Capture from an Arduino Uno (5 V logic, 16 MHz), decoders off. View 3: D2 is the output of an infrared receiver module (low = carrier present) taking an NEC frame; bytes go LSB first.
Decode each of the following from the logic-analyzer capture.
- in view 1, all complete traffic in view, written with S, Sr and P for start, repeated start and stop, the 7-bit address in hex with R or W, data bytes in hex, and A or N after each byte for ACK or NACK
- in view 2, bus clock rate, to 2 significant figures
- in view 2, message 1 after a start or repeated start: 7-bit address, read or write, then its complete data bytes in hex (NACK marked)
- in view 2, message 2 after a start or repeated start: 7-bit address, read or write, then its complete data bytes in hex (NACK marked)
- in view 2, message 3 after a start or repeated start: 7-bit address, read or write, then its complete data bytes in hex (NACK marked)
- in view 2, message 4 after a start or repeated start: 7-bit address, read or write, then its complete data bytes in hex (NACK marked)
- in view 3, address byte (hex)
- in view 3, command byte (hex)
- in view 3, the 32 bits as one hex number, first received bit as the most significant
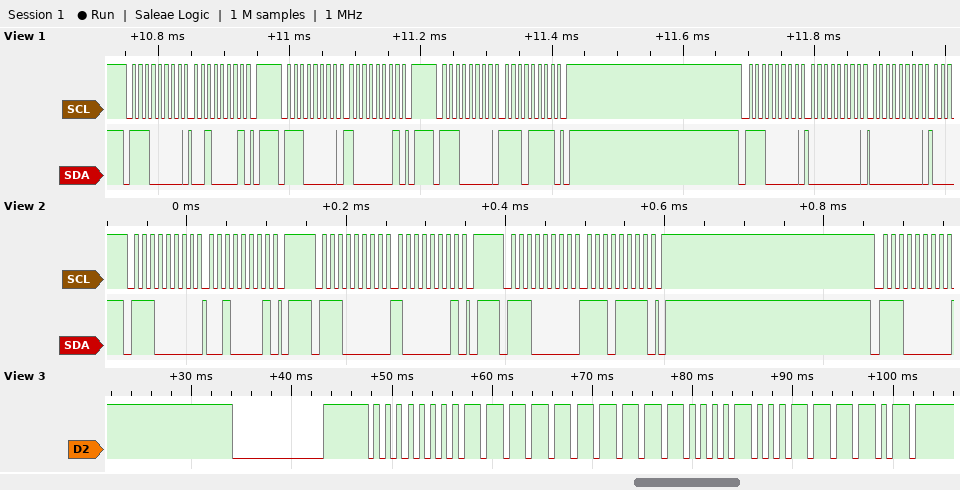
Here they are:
S 70W A 21 A P S 70W A 81 A P S 70W A EF A P S 70W A 00 A 00 A
100 kHz
0x70 write: 21
0x70 write: 81
0x70 write: EF
0x70 write
0x00
0x43
0x00FFC23D
